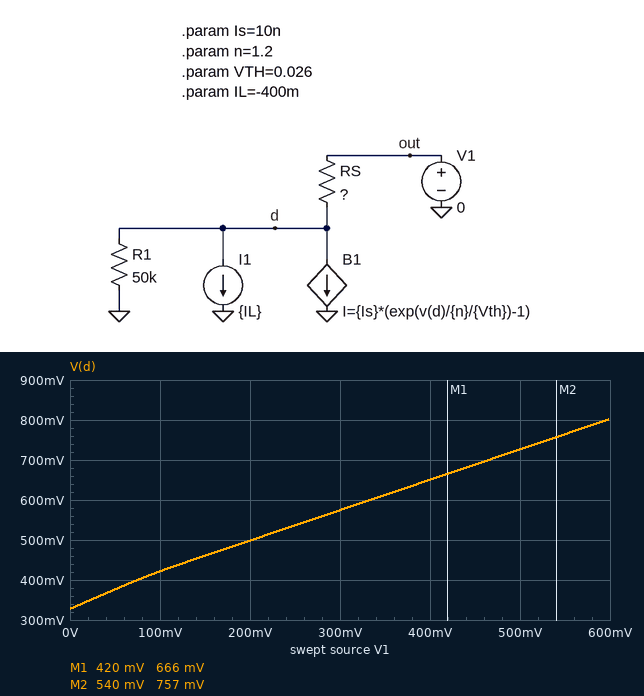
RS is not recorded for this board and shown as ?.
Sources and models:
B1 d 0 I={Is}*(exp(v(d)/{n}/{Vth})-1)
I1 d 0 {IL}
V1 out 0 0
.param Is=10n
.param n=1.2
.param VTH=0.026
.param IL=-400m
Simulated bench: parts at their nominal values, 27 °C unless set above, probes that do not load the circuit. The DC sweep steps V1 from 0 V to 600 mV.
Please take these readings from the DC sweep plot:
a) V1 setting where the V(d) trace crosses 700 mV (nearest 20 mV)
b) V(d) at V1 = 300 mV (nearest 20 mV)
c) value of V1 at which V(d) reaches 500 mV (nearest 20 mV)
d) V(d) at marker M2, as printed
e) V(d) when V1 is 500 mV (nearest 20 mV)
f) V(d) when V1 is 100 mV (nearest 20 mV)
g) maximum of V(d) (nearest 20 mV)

460 mV
580 mV
200 mV
757 mV
720 mV
420 mV
800 mV
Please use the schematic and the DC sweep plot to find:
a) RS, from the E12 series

0.82 Ω
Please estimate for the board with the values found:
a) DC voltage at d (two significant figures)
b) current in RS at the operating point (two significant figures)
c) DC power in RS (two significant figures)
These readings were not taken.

330 mV
400 mA
130 mW
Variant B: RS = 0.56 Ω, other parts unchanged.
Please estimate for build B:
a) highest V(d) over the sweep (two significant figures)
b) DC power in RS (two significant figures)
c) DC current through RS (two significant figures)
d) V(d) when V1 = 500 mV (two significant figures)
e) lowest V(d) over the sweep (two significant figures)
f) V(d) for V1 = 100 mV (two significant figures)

750 mV
90 mW
400 mA
670 mV
220 mV
320 mV
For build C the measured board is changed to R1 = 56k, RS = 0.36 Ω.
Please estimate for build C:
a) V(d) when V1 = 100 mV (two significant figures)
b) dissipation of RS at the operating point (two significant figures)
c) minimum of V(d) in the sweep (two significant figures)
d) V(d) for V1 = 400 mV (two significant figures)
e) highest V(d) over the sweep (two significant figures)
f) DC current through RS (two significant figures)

240 mV
58 mW
140 mV
530 mV
700 mV
400 mA
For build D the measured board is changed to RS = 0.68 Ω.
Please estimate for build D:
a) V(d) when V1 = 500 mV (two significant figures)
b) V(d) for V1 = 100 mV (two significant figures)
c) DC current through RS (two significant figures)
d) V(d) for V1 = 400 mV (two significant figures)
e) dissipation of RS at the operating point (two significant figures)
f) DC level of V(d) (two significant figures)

700 mV
370 mV
400 mA
620 mV
110 mW
270 mV
